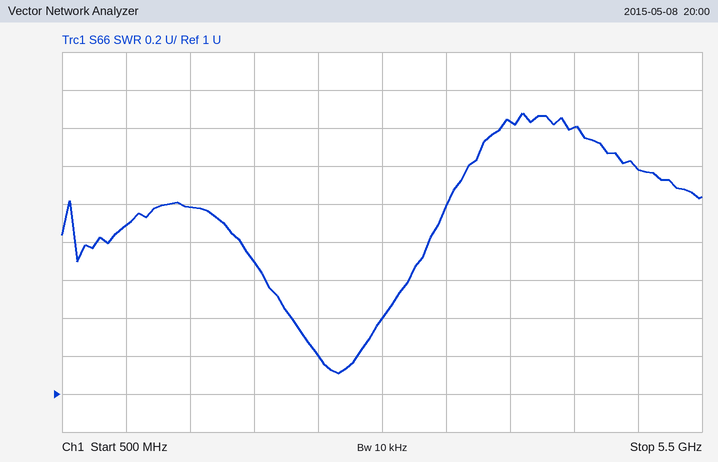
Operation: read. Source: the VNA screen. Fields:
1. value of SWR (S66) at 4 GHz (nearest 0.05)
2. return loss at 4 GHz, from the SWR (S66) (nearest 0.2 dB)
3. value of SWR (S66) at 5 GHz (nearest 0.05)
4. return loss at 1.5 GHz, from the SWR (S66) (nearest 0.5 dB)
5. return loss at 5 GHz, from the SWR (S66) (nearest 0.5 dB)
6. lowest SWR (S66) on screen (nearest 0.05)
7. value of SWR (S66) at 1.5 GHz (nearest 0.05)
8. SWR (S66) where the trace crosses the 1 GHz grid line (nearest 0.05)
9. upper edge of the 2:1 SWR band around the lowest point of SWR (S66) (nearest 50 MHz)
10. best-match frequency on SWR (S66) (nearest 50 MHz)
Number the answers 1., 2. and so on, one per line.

1. 2.45
2. 7.6 dB
3. 2.20
4. 9.5 dB
5. 8.5 dB
6. 1.10
7. 2.00
8. 1.90
9. 3.50 GHz
10. 2.65 GHz
